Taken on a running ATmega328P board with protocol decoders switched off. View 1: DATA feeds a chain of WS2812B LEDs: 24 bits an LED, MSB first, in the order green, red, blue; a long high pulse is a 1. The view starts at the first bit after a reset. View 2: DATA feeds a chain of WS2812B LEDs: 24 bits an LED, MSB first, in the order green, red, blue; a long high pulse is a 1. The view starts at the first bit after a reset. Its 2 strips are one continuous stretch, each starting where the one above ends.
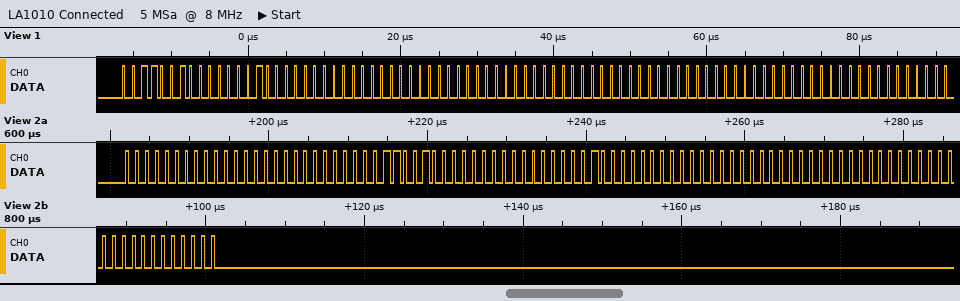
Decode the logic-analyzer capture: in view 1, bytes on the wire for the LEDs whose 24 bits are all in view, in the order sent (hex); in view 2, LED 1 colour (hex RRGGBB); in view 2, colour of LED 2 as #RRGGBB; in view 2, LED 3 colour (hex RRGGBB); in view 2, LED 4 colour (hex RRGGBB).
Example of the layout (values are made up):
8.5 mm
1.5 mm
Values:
32 02 00 00 00 00 00 00 00
#000000
#003201
#000000
#000000
